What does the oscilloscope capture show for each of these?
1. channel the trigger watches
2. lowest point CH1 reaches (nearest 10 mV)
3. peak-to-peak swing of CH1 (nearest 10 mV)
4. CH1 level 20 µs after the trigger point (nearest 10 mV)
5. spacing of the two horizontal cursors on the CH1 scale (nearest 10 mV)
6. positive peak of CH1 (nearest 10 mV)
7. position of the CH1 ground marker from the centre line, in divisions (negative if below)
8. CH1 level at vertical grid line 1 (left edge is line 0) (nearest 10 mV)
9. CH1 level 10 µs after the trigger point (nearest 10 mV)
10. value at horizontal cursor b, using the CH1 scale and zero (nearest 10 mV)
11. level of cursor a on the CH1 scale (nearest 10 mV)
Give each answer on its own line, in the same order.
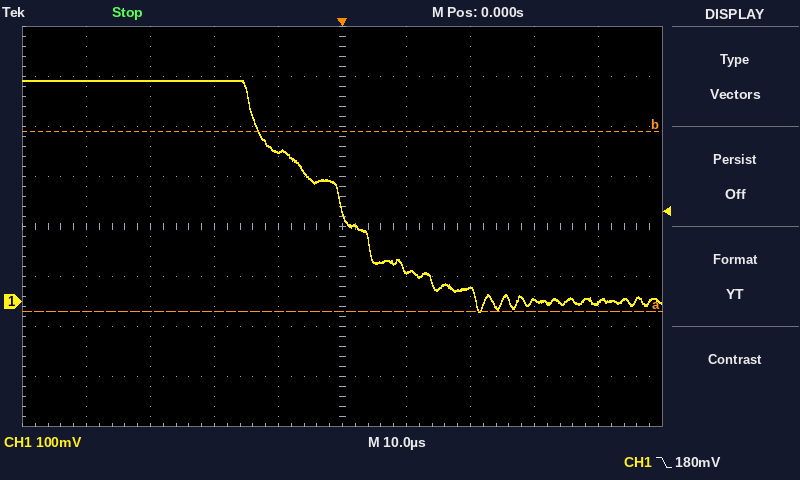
CH1
-20 mV
460 mV
30 mV
360 mV
440 mV
-1.5 div
440 mV
60 mV
340 mV
-20 mV
